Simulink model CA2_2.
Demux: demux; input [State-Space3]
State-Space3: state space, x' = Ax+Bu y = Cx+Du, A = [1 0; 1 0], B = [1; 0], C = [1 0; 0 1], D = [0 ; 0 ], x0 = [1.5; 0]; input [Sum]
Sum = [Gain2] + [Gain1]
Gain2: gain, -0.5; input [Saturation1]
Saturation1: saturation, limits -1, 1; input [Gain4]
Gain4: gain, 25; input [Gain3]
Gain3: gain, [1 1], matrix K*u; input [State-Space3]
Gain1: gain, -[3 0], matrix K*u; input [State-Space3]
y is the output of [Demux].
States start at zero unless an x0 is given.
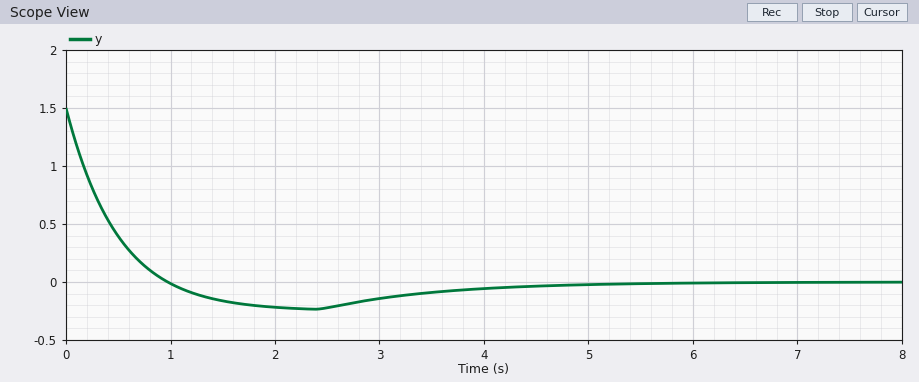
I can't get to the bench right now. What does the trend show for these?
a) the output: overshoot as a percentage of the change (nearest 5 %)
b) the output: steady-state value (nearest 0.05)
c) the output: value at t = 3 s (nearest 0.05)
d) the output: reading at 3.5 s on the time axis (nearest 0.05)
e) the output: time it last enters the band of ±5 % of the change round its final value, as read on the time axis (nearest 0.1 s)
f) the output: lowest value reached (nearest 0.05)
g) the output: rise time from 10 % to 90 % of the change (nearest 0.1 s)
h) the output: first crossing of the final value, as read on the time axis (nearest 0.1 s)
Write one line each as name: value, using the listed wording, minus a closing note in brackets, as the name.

the output: overshoot as a percentage of the change: 15 %
the output: steady-state value: 0.00
the output: value at t = 3 s: -0.15
the output: reading at 3.5 s on the time axis: -0.10
the output: time it last enters the band of ±5 % of the change round its final value, as read on the time axis: 3.7 s
the output: lowest value reached: -0.25
the output: rise time from 10 % to 90 % of the change: 0.7 s
the output: first crossing of the final value, as read on the time axis: 1.0 s
